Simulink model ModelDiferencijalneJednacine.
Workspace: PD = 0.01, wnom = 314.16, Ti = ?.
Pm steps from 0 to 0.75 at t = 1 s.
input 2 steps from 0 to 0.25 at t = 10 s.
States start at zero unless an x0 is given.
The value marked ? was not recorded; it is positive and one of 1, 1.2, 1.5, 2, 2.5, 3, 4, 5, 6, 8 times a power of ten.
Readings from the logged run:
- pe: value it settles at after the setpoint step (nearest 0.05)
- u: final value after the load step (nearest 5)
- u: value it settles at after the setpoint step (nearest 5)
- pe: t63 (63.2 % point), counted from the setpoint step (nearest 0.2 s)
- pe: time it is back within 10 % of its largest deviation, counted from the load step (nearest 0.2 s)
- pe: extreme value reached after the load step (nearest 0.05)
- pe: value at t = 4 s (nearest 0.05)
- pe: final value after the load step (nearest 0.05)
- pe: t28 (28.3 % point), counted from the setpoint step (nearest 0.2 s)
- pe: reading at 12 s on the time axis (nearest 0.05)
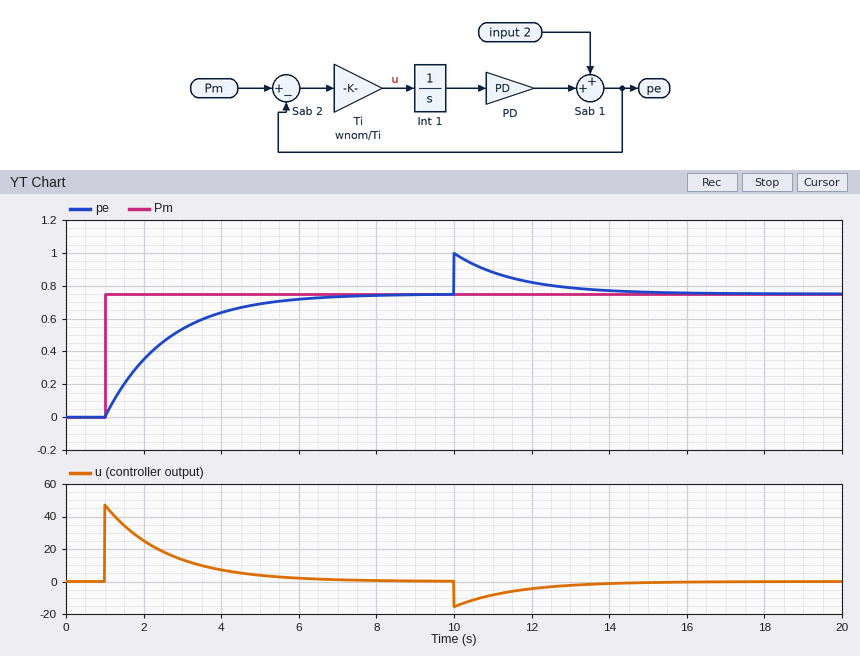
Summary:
0.75
0
0
1.6 s
3.6 s
1.00
0.65
0.75
0.6 s
0.80
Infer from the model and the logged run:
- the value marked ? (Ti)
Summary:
5
